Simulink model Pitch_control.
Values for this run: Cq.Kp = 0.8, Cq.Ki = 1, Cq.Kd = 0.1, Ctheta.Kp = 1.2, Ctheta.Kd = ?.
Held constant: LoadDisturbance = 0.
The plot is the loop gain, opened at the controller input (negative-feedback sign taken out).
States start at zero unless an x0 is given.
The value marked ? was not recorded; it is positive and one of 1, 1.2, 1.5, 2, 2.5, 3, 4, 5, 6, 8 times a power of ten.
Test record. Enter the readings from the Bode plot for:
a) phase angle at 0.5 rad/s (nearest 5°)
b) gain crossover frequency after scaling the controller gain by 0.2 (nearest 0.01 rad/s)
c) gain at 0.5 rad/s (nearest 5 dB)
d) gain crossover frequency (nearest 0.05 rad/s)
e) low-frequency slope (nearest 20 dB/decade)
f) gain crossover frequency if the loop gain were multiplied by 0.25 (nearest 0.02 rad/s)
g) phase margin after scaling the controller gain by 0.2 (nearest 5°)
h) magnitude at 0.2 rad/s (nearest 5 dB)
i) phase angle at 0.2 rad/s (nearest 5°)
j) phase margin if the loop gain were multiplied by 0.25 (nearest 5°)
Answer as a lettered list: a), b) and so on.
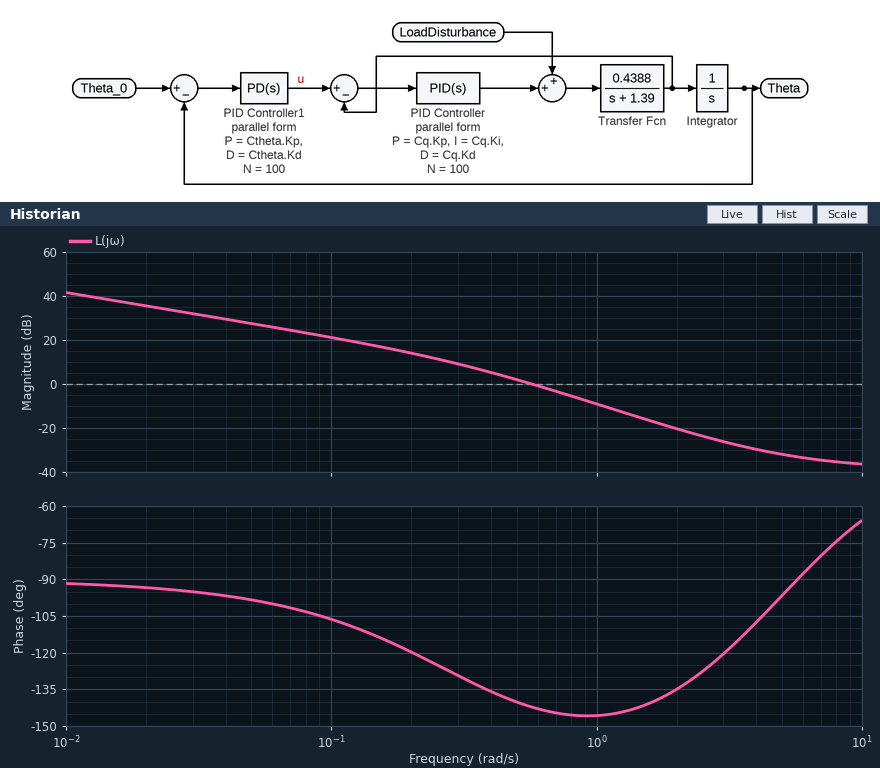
a) -140°
b) 0.20 rad/s
c) 0 dB
d) 0.55 rad/s
e) -20 dB/decade
f) 0.24 rad/s
g) 60°
h) 15 dB
i) -120°
j) 55°
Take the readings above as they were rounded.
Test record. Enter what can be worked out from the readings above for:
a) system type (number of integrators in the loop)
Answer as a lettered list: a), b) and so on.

a) 1
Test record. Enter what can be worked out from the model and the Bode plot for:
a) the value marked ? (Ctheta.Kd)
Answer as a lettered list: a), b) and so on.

a) 0.25
